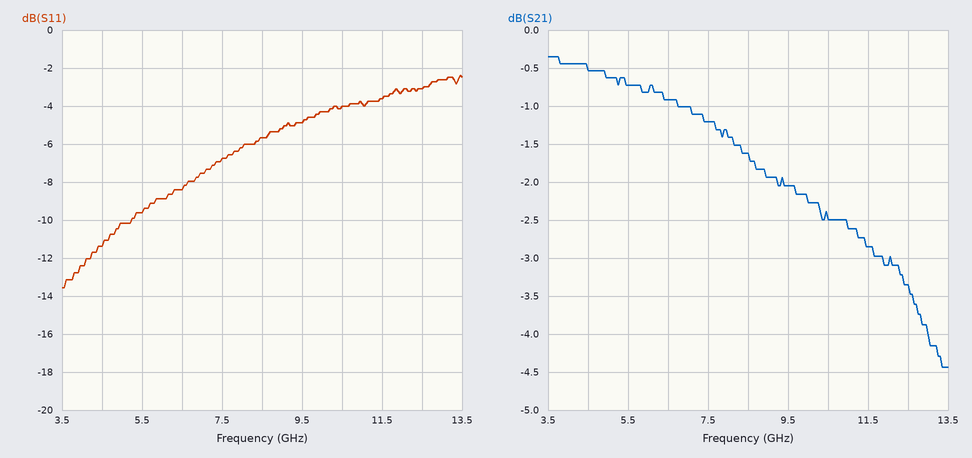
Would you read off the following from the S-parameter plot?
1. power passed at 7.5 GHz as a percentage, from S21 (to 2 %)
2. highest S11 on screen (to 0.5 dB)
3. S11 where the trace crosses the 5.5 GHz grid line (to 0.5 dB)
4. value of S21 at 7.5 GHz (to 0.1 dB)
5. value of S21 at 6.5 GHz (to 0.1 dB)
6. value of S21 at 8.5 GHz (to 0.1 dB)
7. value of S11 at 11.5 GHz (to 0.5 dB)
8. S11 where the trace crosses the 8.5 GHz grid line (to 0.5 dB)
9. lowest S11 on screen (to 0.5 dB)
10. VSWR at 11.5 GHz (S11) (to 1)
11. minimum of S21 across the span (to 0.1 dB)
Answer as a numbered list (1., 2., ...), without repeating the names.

1. 76 %
2. -2.5 dB
3. -9.5 dB
4. -1.2 dB
5. -0.9 dB
6. -1.6 dB
7. -3.5 dB
8. -5.5 dB
9. -13.5 dB
10. 5
11. -4.4 dB
